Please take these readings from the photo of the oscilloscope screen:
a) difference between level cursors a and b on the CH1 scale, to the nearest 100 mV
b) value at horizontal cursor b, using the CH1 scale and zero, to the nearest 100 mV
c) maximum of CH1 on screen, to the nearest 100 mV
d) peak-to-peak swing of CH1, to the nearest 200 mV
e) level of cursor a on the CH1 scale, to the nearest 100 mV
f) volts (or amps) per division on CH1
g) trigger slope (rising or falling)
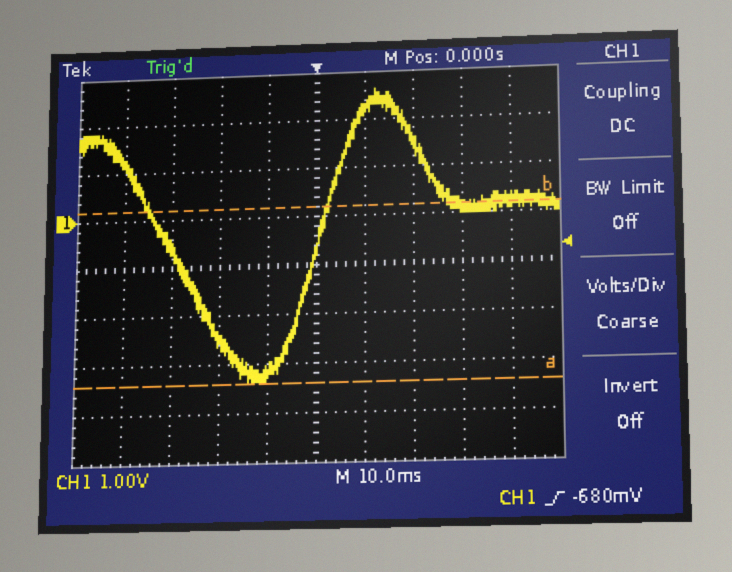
3.6 V
200 mV
2.6 V
6.0 V
-3.4 V
1 V
rising
